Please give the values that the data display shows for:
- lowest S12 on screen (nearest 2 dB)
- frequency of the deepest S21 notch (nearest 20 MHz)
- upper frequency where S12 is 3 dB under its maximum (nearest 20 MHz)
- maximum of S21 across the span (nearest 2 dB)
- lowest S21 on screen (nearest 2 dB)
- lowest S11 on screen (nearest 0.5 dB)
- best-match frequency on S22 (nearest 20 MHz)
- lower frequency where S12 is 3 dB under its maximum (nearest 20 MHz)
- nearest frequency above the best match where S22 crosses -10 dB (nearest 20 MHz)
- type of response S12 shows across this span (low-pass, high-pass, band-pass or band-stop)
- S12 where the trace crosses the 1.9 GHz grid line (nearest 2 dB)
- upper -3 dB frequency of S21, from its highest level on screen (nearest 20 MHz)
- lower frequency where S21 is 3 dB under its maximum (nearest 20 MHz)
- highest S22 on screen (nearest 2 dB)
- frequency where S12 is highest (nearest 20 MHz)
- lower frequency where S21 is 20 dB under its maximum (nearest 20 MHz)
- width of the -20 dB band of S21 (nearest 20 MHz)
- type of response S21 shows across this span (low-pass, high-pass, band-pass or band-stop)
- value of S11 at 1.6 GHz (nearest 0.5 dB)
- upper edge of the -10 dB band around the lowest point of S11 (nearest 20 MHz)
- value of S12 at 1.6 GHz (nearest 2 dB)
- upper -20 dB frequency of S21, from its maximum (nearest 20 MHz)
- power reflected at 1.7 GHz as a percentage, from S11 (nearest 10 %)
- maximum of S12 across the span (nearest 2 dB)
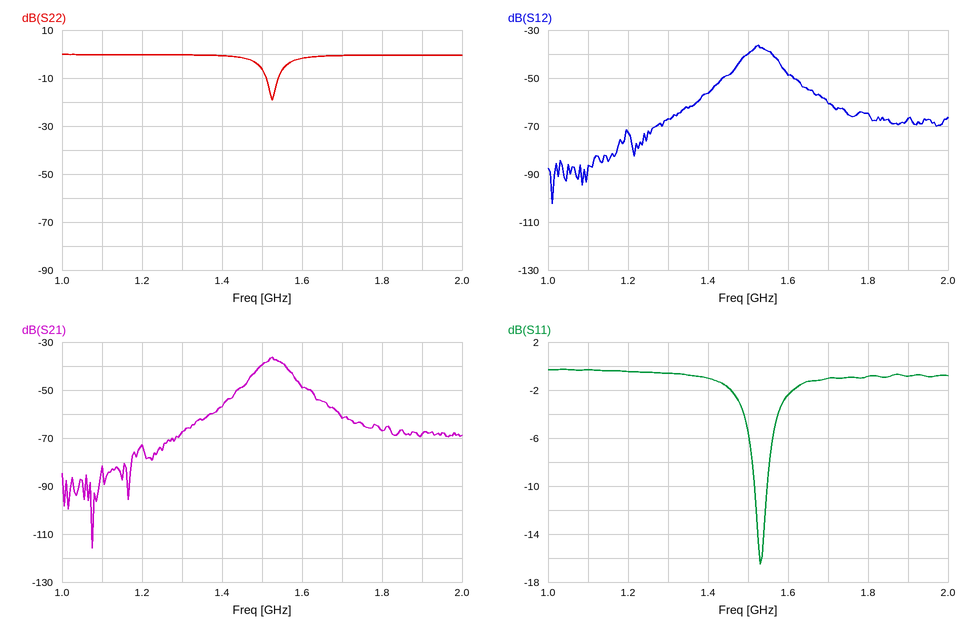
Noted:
-102 dB
1.08 GHz
1.56 GHz
-36 dB
-116 dB
-16.5 dB
1.52 GHz
1.50 GHz
1.54 GHz
band-pass
-66 dB
1.56 GHz
1.50 GHz
0 dB
1.52 GHz
1.40 GHz
260 MHz
band-pass
-2.5 dB
1.54 GHz
-48 dB
1.66 GHz
80 %
-36 dB
